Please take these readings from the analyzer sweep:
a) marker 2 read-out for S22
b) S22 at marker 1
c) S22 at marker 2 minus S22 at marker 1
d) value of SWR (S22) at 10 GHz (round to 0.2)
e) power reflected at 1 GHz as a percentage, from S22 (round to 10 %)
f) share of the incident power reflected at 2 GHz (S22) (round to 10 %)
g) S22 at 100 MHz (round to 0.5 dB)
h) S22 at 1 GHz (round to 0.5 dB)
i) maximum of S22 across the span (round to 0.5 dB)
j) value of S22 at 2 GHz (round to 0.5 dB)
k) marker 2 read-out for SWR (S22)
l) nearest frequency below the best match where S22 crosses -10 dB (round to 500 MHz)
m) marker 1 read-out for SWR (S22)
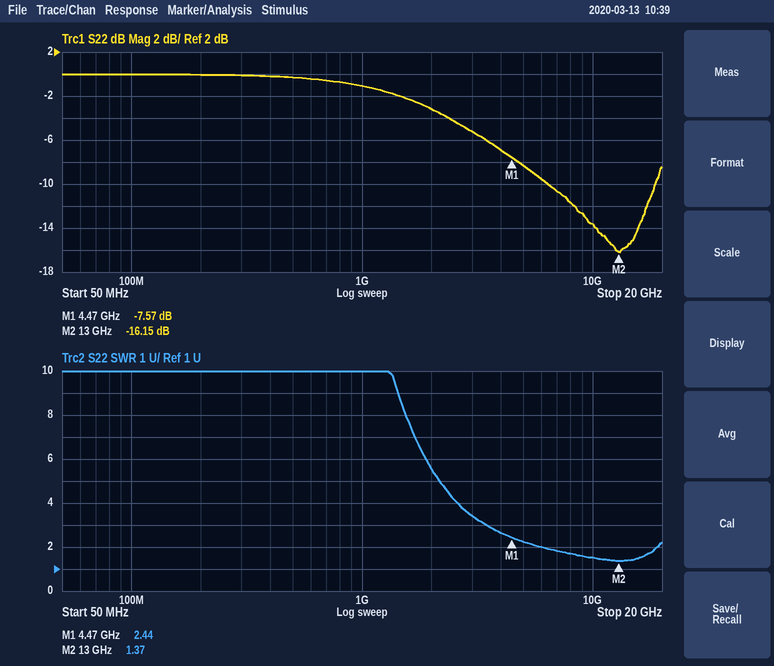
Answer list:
-16.15 dB
-7.57 dB
-8.58 dB
1.6
80 %
50 %
0.0 dB
-1.0 dB
0.0 dB
-3.0 dB
1.37
6.5 GHz
2.44
